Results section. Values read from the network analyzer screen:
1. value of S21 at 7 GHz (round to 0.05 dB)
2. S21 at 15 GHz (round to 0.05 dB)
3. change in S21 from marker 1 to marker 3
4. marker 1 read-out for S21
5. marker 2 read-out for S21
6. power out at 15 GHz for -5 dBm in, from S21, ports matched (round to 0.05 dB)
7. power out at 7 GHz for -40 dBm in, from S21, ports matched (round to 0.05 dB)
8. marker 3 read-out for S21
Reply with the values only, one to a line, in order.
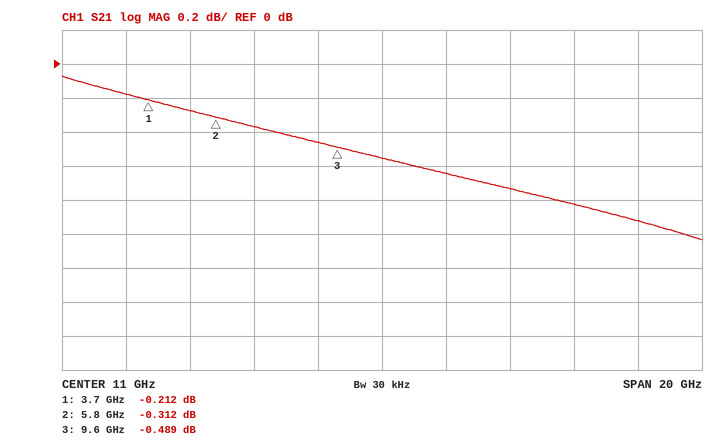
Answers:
-0.35 dB
-0.75 dB
-0.277 dB
-0.212 dB
-0.312 dB
-5.75 dBm
-40.35 dBm
-0.489 dB
